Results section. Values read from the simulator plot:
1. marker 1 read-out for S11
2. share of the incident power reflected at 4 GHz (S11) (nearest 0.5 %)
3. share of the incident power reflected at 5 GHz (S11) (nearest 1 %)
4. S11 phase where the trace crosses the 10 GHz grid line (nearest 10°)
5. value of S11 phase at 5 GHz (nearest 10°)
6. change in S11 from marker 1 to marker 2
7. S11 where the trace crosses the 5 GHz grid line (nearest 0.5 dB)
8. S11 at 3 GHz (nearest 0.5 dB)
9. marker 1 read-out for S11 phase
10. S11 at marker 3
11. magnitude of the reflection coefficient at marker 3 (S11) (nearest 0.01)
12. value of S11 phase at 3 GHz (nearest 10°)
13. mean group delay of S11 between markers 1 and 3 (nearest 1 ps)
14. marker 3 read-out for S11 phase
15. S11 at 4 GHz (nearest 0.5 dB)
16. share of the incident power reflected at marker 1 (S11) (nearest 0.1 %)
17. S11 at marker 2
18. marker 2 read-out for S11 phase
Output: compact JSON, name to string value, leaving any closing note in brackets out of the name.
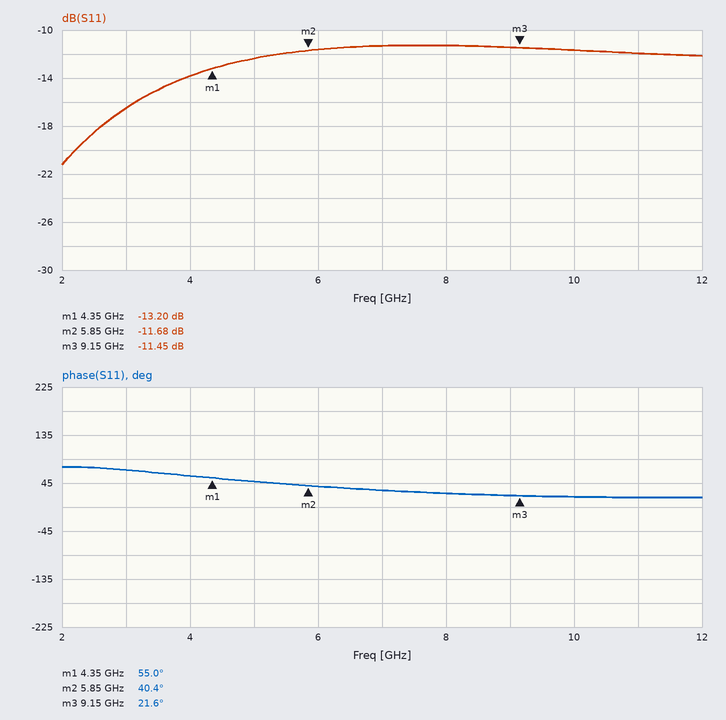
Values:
{"marker 1 read-out for S11": "-13.20 dB", "share of the incident power reflected at 4 GHz (S11)": "4.0 %", "share of the incident power reflected at 5 GHz (S11)": "6 %", "S11 phase where the trace crosses the 10 GHz grid line": "20°", "value of S11 phase at 5 GHz": "50°", "change in S11 from marker 1 to marker 2": "1.52 dB", "S11 where the trace crosses the 5 GHz grid line": "-12.5 dB", "S11 at 3 GHz": "-16.5 dB", "marker 1 read-out for S11 phase": "55.0°", "S11 at marker 3": "-11.45 dB", "magnitude of the reflection coefficient at marker 3 (S11)": "0.27", "value of S11 phase at 3 GHz": "70°", "mean group delay of S11 between markers 1 and 3": "19 ps", "marker 3 read-out for S11 phase": "21.6°", "S11 at 4 GHz": "-14.0 dB", "share of the incident power reflected at marker 1 (S11)": "4.8 %", "S11 at marker 2": "-11.68 dB", "marker 2 read-out for S11 phase": "40.4°"}
